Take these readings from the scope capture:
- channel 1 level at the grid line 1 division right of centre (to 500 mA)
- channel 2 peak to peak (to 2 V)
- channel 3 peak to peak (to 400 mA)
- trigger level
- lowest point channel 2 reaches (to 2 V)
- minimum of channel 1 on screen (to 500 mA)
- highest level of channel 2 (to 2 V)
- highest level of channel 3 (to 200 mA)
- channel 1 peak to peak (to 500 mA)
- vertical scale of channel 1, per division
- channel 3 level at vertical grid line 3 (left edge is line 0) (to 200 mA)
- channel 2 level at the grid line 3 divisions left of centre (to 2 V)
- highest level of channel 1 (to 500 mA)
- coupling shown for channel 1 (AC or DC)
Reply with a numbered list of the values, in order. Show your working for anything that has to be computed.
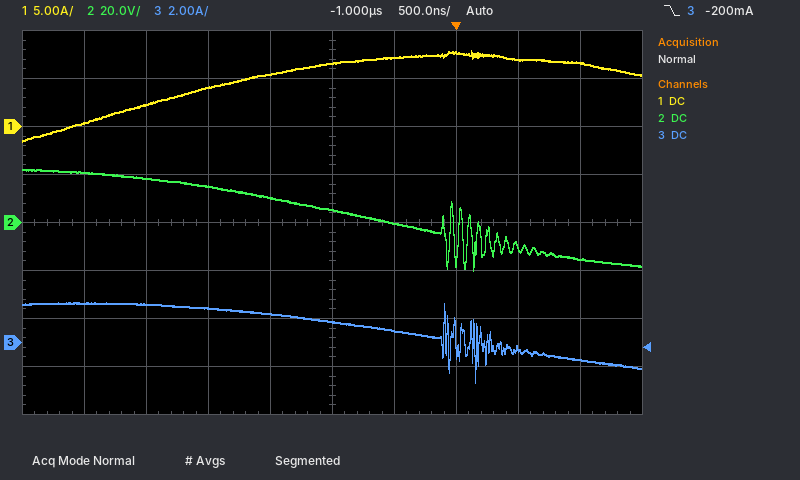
1. 7.0 A
2. 22 V − (-20 V) = 42 V
3. 3.2 A
4. -200 mA
5. -20 V
6. -1.5 A
7. 22 V
8. 1.6 A
9. 8.0 A − (-1.5 A) = 9.5 A
10. 5 A
11. 1.4 A
12. 18 V
13. 8.0 A
14. DC
